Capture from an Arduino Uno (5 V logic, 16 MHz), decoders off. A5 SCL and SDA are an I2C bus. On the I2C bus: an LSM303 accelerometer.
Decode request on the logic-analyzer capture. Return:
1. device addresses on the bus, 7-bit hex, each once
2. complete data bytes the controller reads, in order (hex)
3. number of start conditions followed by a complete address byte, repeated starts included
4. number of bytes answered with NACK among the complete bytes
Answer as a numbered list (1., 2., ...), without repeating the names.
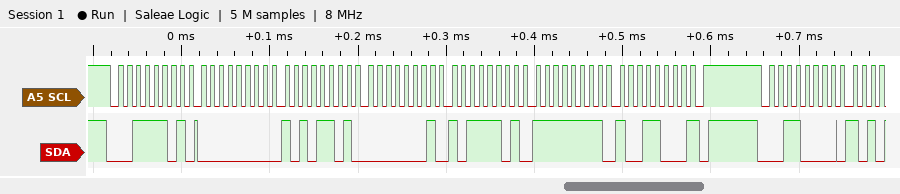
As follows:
1. 0x1E 0x18
2. 00 AD 01 BD FF 98
3. 2
4. 1
